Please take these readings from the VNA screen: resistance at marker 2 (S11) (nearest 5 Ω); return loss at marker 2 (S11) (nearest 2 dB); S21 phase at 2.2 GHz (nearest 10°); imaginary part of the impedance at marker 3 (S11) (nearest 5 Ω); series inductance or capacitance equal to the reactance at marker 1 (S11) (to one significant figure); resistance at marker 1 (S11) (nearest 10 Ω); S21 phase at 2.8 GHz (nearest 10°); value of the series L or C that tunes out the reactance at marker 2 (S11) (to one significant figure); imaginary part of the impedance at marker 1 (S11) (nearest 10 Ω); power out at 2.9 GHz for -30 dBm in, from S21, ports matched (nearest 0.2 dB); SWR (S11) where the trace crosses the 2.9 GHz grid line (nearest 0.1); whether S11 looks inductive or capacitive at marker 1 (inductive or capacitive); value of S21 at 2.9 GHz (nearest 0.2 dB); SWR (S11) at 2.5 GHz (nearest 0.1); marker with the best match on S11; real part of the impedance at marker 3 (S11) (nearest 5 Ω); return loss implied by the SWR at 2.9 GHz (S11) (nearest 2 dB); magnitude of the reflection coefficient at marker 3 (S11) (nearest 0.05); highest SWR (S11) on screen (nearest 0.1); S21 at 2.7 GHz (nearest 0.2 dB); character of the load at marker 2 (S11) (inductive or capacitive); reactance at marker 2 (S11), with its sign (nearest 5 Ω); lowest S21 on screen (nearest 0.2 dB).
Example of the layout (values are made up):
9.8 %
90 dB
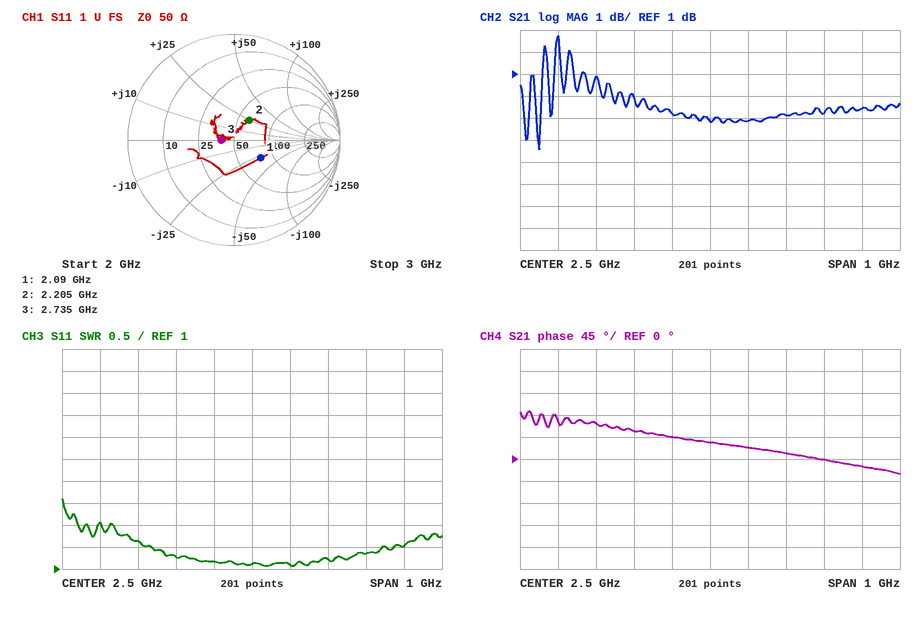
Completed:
60 Ω
12 dB
70°
0 Ω
3 pF
80 Ω
0°
3 pF
-30 Ω
-30.6 dBm
1.5
capacitive
-0.6 dB
1.1
marker 3
40 Ω
14 dB
0.10
2.6
-0.8 dB
inductive
+25 Ω
-2.4 dB
